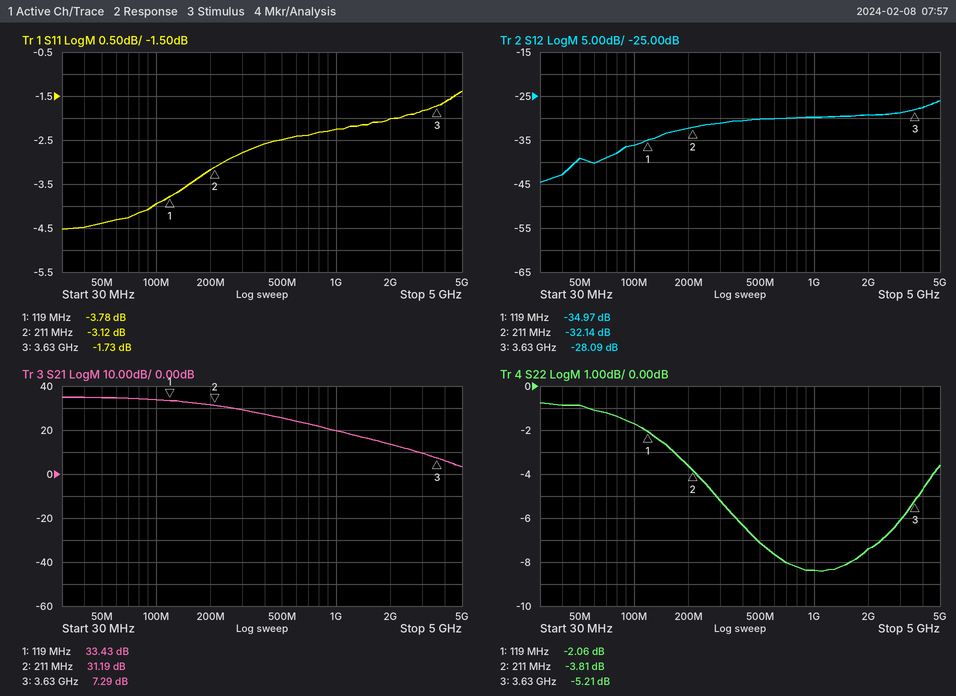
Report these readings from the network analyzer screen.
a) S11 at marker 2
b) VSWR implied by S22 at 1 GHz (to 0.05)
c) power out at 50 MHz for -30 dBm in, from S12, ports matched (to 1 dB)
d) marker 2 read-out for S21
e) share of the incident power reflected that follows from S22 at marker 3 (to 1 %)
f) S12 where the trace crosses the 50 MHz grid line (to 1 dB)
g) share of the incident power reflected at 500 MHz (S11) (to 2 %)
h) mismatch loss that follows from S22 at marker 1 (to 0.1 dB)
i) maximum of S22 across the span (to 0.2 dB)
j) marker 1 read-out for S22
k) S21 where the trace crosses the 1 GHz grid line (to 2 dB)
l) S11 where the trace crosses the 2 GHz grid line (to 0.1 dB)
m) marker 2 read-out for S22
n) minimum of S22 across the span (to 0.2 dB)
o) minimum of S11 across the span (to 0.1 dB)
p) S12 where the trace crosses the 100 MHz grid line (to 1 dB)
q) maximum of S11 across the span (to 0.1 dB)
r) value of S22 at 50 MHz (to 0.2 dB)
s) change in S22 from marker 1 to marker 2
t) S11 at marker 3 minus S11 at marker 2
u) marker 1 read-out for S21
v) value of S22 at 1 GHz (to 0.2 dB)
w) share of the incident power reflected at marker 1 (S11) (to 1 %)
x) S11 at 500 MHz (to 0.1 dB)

-3.12 dB
2.25
-69 dBm
31.19 dB
30 %
-39 dB
56 %
4.2 dB
-0.8 dB
-2.06 dB
20 dB
-2.0 dB
-3.81 dB
-8.4 dB
-4.5 dB
-36 dB
-1.4 dB
-0.8 dB
-1.75 dB
1.39 dB
33.43 dB
-8.4 dB
42 %
-2.5 dB
